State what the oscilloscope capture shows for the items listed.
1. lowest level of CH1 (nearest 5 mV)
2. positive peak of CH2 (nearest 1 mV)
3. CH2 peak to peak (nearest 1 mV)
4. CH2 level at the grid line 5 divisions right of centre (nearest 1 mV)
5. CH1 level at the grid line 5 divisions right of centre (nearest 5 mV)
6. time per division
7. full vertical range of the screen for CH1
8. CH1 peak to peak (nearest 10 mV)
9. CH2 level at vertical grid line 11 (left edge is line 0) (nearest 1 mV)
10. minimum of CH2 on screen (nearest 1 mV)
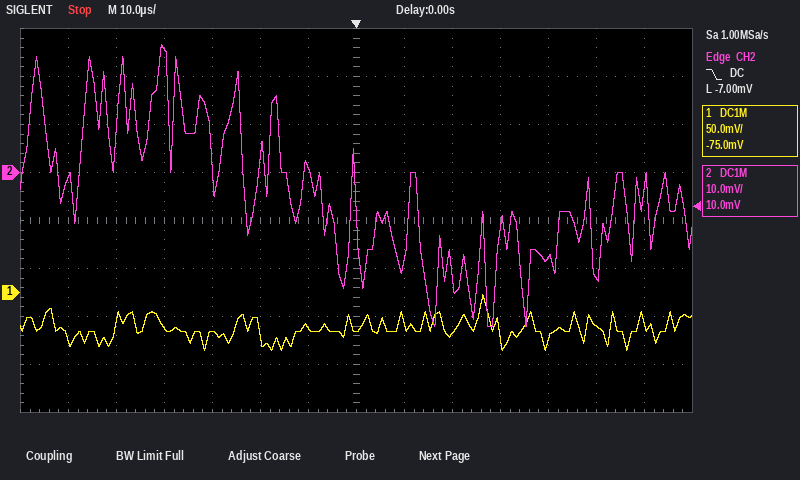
-60 mV
27 mV
59 mV
-22 mV
-35 mV
10 µs
400 mV
60 mV
-18 mV
-32 mV
